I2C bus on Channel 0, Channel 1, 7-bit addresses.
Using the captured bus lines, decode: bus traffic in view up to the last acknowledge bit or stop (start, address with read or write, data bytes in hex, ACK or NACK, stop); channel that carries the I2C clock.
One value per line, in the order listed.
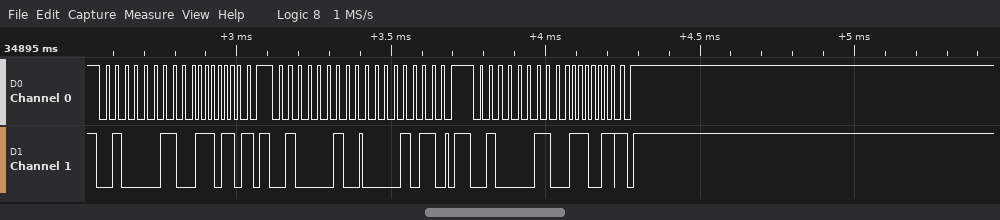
start, address 21 read ACK, 76 NACK, stop, start, address 21 write ACK, 0B ACK, stop, start, address 21 read ACK, 73 NACK, stop
Channel 0
